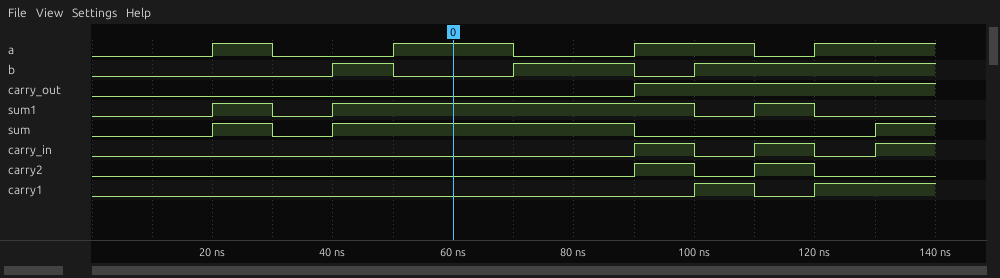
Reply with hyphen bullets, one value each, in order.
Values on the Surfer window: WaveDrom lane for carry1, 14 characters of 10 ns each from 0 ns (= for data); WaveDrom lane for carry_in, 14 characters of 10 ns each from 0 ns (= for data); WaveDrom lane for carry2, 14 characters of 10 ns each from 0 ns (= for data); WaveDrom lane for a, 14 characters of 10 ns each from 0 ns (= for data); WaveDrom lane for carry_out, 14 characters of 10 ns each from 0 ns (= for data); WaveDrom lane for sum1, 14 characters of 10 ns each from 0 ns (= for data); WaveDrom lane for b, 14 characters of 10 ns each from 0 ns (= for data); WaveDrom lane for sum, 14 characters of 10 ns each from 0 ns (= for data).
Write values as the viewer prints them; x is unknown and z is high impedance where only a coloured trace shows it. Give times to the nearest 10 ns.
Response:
- {name: 'carry1', wave: '0.........101.'}
- {name: 'carry_in', wave: '0........10101'}
- {name: 'carry2', wave: '0........1010.'}
- {name: 'a', wave: '0.10.1.0.1.01.'}
- {name: 'carry_out', wave: '0........1....'}
- {name: 'sum1', wave: '0.101.....010.'}
- {name: 'b', wave: '0...10.1.01...'}
- {name: 'sum', wave: '0.101....0...1'}
